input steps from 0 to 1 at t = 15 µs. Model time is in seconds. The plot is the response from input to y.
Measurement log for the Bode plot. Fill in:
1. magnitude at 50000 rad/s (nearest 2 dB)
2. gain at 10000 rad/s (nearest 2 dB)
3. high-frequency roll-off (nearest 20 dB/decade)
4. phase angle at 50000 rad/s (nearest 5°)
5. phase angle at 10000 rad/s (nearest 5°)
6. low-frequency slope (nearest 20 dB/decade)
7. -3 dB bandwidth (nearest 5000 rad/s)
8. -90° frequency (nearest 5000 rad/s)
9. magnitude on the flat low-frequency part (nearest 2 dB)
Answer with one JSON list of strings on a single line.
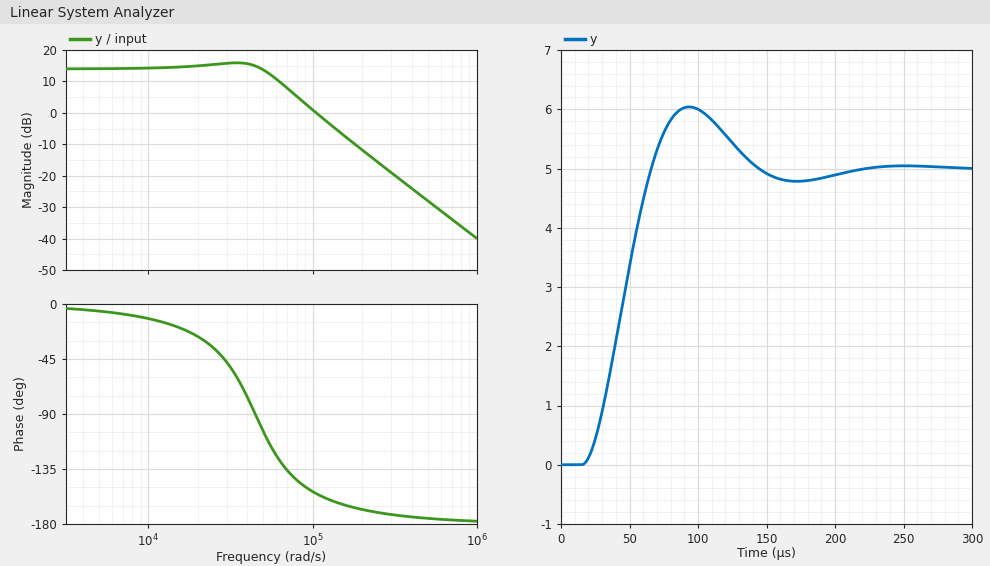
["14 dB", "14 dB", "-40 dB/decade", "-105°", "-10°", "0 dB/decade", "60000 rad/s", "45000 rad/s", "14 dB"]
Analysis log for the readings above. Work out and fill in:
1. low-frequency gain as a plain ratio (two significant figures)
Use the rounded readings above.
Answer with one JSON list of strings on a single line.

["5.0"]
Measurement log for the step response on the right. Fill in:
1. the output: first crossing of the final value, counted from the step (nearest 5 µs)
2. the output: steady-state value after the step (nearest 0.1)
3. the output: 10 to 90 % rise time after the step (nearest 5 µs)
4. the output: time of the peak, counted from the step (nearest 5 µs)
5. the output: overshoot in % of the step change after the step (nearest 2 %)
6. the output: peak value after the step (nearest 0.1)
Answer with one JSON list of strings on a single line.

["50 µs", "5.0", "35 µs", "80 µs", "20 %", "6.0"]
